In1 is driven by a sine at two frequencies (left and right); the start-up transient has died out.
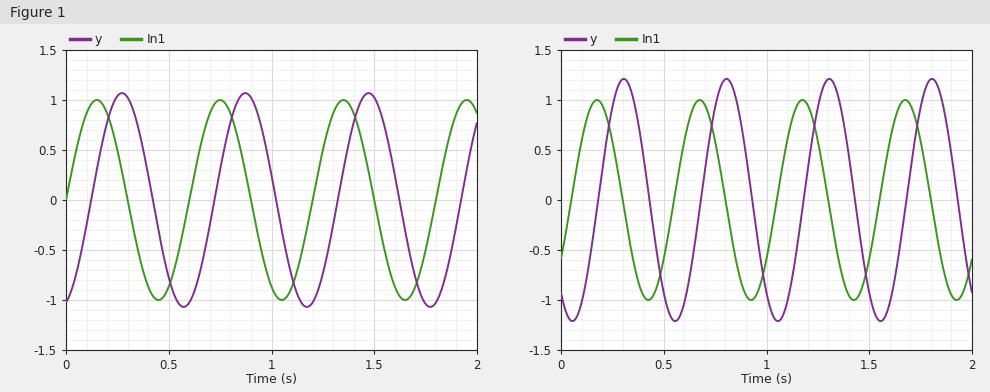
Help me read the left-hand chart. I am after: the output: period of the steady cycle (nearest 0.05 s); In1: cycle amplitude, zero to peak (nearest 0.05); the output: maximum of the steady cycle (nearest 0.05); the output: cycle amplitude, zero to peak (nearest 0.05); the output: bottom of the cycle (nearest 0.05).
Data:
0.60 s
1.00
1.05
1.05
-1.05
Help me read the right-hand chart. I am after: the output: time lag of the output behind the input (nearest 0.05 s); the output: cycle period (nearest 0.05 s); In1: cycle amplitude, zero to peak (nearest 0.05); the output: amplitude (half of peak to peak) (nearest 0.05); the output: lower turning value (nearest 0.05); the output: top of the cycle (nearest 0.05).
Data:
0.15 s
0.50 s
1.00
1.20
-1.20
1.20
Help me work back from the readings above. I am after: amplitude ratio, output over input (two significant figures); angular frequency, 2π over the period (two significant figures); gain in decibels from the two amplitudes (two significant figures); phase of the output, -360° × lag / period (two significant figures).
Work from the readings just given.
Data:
1.2
13 rad/s
1.6 dB
-110°
